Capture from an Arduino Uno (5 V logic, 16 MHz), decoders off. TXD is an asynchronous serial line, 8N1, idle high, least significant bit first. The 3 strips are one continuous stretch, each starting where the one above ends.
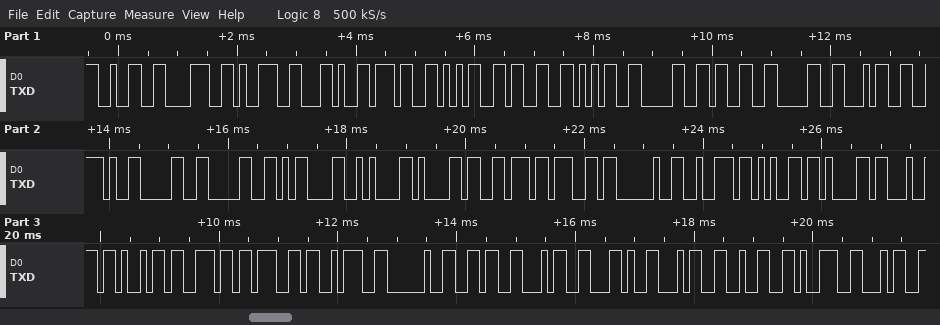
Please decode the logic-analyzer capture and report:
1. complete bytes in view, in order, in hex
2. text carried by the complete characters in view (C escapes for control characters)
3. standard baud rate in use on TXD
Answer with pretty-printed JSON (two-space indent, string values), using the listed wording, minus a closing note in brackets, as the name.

{
  "complete bytes in view, in order, in hex": "32 38 39 2C 37 35 33 35 30 33 30 34 2E 30 30 0D 0A 61 76 67 20 72 65 61 64 69 6E 67 3A 20 36 34 2C 34 32 39 34",
  "text carried by the complete characters in view": "\"289,75350304.00\\r\\navg reading: 64,4294\"",
  "standard baud rate in use on TXD": "9600 baud"
}
